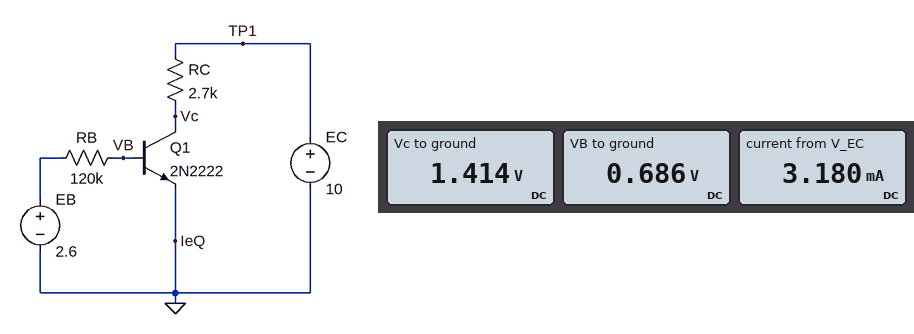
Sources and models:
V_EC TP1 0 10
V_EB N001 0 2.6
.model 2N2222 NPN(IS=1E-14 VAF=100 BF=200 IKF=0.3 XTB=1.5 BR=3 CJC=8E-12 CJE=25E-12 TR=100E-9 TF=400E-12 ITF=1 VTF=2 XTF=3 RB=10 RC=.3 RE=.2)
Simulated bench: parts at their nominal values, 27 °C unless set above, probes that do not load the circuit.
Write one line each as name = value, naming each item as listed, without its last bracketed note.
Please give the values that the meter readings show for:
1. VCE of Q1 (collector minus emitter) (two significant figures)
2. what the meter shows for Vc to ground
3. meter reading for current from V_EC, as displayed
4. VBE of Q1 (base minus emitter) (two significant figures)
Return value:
VCE of Q1 (collector minus emitter) = 1.4 V
what the meter shows for Vc to ground = 1.414 V
meter reading for current from V_EC, as displayed = 3.180 mA
VBE of Q1 (base minus emitter) = 690 mV
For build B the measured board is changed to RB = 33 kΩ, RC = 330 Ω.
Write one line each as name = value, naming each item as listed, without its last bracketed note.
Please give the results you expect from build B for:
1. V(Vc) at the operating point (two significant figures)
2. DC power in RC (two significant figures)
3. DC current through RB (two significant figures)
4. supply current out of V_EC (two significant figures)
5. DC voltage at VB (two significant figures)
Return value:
V(Vc) at the operating point = 6.2 V
DC power in RC = 44 mW
DC current through RB = 57 µA
supply current out of V_EC = 12 mA
DC voltage at VB = 720 mV
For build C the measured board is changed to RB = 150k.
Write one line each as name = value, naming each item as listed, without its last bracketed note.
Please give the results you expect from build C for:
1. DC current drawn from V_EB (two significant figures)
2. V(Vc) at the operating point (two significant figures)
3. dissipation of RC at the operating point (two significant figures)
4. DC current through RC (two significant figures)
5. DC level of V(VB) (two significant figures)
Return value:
DC current drawn from V_EB = 13 µA
V(Vc) at the operating point = 3.0 V
dissipation of RC at the operating point = 18 mW
DC current through RC = 2.6 mA
DC level of V(VB) = 680 mV
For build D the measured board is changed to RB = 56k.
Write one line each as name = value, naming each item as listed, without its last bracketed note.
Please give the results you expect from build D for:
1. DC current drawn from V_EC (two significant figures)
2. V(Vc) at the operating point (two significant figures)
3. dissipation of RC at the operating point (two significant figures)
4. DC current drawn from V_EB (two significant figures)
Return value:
DC current drawn from V_EC = 3.7 mA
V(Vc) at the operating point = 120 mV
dissipation of RC at the operating point = 36 mW
DC current drawn from V_EB = 34 µA
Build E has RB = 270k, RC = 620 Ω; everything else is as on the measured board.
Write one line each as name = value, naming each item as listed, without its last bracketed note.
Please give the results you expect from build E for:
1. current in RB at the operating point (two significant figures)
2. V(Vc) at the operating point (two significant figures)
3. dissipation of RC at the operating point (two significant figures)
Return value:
current in RB at the operating point = 7.2 µA
V(Vc) at the operating point = 9.0 V
dissipation of RC at the operating point = 1.5 mW
